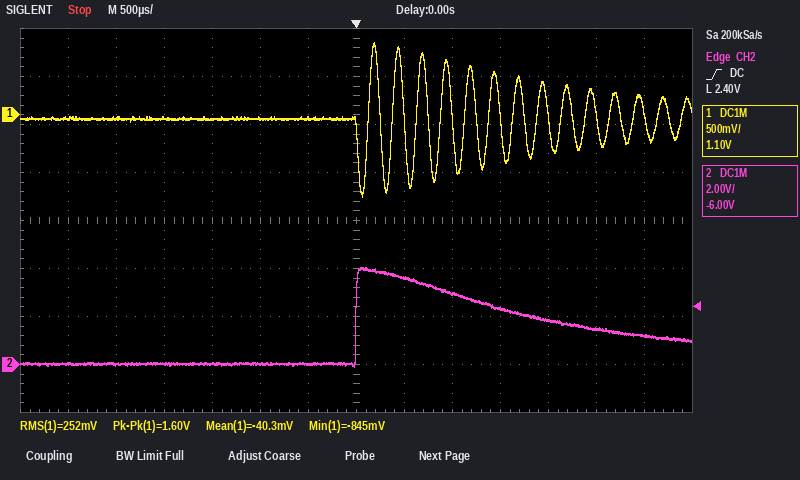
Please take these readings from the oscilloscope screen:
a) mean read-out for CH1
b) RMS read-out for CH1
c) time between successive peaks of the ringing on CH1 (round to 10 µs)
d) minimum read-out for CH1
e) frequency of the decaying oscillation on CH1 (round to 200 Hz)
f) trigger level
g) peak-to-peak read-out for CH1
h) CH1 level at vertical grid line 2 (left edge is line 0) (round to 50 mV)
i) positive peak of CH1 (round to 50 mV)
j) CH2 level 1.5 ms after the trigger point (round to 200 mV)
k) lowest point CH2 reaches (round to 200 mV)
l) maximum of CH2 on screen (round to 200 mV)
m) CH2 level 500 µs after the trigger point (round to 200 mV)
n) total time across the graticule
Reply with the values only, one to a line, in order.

-40.3 mV
252 mV
250 µs
-845 mV
4.0 kHz
2.40 V
1.60 V
-50 mV
750 mV
2.4 V
0.0 V
4.0 V
3.6 V
7 ms
